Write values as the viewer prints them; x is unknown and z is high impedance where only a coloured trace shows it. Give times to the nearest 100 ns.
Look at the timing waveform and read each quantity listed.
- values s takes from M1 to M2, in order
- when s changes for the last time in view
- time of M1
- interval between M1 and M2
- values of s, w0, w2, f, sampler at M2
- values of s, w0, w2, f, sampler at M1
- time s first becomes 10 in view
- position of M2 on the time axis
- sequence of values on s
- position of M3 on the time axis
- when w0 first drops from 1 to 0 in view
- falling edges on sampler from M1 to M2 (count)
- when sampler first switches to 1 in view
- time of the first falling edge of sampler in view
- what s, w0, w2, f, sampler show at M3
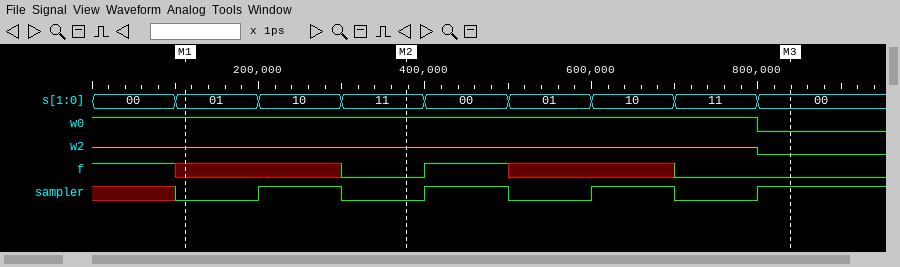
01, 10, 11
800 ns
100 ns
300 ns
s=11, w0=1, w2=z, f=0, sampler=0
s=01, w0=1, w2=z, f=x, sampler=0
200 ns
400 ns
00, 01, 10, 11, 00, 01, 10, 11, 00
800 ns
800 ns
1
200 ns
300 ns
s=00, w0=0, w2=0, f=0, sampler=1
